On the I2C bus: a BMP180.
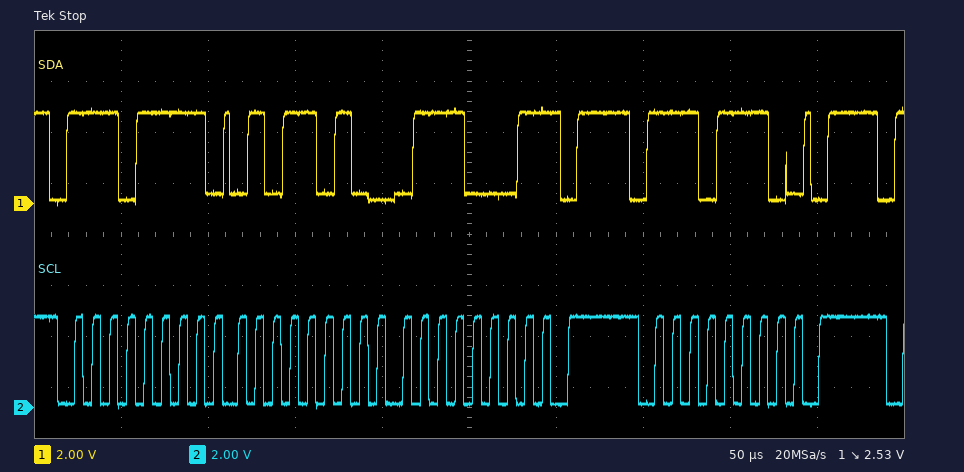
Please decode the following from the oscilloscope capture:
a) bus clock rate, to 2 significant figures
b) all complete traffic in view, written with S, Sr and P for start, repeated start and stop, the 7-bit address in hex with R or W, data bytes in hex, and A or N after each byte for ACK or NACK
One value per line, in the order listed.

100 kHz
S 77R A 5A A 71 N P S 77W A P
